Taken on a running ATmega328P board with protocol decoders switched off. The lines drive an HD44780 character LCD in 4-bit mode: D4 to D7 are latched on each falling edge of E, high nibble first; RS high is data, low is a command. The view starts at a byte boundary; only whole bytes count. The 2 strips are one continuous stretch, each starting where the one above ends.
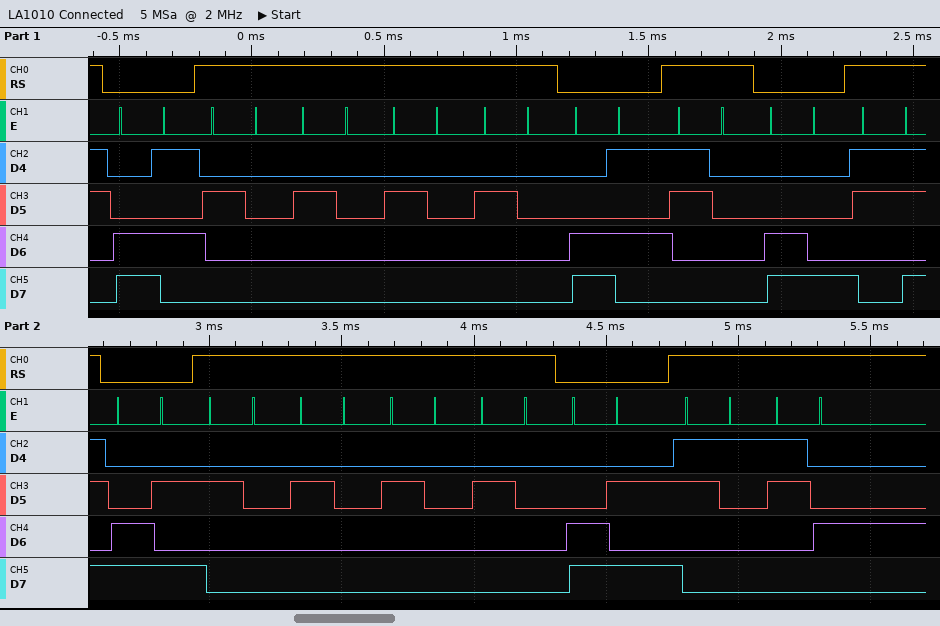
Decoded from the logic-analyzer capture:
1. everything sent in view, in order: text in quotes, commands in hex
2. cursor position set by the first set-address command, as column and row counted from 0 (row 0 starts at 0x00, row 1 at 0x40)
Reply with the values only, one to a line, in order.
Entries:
0xC5 "    " 0xC5 "0" 0xC8 ";" 0xCA "    " 0xCA "14"
column 5, row 1
